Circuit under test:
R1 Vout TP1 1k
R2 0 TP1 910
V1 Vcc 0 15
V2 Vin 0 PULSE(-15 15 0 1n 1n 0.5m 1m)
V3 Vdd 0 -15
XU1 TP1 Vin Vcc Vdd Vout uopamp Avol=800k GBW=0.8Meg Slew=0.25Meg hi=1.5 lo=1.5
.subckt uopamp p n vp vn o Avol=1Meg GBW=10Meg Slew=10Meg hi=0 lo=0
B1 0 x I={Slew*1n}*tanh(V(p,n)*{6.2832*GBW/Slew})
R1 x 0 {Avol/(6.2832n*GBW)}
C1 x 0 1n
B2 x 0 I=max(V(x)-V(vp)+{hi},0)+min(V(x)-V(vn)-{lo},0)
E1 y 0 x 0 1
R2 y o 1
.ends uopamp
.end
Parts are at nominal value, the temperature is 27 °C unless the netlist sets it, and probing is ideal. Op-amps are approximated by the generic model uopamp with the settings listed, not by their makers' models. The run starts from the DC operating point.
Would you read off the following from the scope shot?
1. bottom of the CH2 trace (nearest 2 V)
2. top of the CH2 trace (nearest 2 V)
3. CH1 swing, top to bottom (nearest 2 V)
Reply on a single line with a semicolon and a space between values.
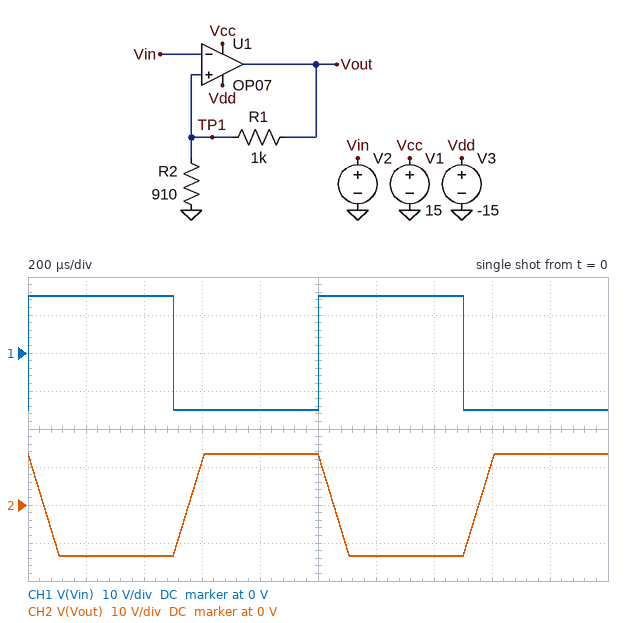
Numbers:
-14 V; 14 V; 30 V
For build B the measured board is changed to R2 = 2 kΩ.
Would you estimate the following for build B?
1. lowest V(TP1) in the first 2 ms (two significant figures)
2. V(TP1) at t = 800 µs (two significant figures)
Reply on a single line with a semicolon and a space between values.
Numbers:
-9.0 V; 9.0 V
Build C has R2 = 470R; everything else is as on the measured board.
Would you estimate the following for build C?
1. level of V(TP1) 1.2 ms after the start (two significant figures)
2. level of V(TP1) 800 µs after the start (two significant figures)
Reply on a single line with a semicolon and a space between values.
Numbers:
-4.3 V; 4.3 V
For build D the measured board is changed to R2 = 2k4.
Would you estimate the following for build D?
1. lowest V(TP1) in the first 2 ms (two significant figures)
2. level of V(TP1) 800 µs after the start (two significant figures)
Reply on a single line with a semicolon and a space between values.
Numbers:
-9.5 V; 9.5 V
